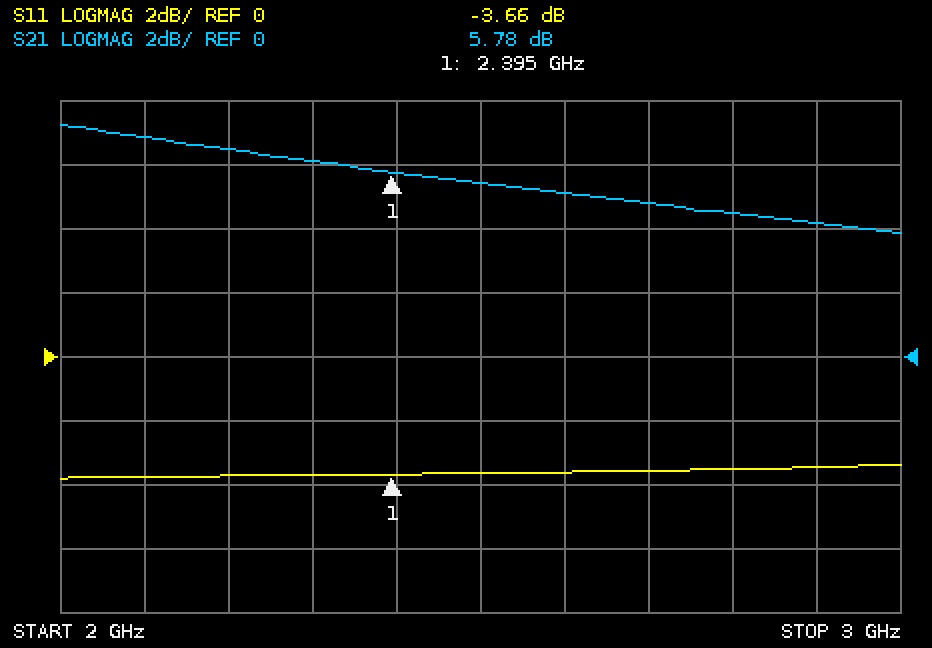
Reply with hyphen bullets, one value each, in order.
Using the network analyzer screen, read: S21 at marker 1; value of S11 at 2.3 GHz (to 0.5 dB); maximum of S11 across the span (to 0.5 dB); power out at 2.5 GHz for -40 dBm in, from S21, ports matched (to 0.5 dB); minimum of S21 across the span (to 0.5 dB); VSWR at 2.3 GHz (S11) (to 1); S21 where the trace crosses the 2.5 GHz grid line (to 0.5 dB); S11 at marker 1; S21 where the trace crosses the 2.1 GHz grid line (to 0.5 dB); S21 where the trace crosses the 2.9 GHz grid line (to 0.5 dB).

- 5.78 dB
- -3.5 dB
- -3.5 dB
- -34.5 dBm
- 4.0 dB
- 5
- 5.5 dB
- -3.66 dB
- 7.0 dB
- 4.0 dB
